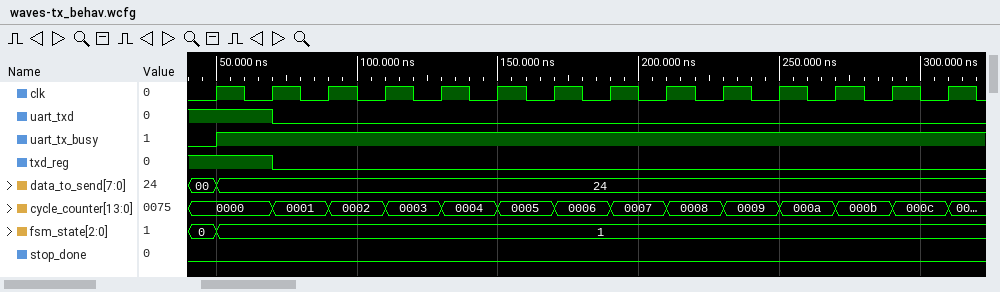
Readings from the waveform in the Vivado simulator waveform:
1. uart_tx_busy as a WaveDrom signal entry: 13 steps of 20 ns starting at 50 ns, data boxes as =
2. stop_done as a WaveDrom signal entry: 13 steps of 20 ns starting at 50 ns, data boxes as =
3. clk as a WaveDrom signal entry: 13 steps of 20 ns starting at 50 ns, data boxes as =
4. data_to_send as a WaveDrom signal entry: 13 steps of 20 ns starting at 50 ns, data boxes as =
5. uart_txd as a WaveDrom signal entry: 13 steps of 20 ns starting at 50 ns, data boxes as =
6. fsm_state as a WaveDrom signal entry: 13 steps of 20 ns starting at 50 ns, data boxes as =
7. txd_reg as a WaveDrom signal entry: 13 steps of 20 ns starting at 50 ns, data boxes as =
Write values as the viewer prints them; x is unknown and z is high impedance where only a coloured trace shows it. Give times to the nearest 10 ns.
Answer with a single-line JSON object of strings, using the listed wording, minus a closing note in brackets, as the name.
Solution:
{"uart_tx_busy as a WaveDrom signal entry: 13 steps of 20 ns starting at 50 ns, data boxes as =": "{name: 'uart_tx_busy', wave: '1............'}", "stop_done as a WaveDrom signal entry: 13 steps of 20 ns starting at 50 ns, data boxes as =": "{name: 'stop_done', wave: '0............'}", "clk as a WaveDrom signal entry: 13 steps of 20 ns starting at 50 ns, data boxes as =": "{name: 'clk', wave: 'p............'}", "data_to_send as a WaveDrom signal entry: 13 steps of 20 ns starting at 50 ns, data boxes as =": "{name: 'data_to_send', wave: '=............', data: '24'}", "uart_txd as a WaveDrom signal entry: 13 steps of 20 ns starting at 50 ns, data boxes as =": "{name: 'uart_txd', wave: '10...........'}", "fsm_state as a WaveDrom signal entry: 13 steps of 20 ns starting at 50 ns, data boxes as =": "{name: 'fsm_state', wave: '=............', data: '1'}", "txd_reg as a WaveDrom signal entry: 13 steps of 20 ns starting at 50 ns, data boxes as =": "{name: 'txd_reg', wave: '10...........'}"}
